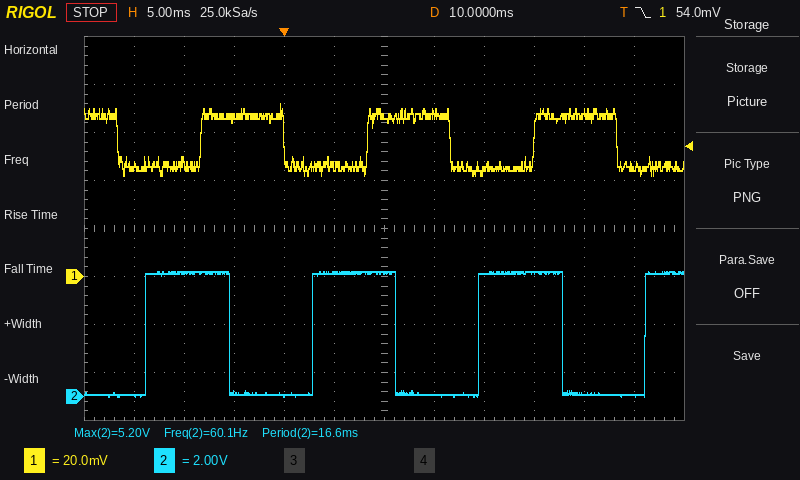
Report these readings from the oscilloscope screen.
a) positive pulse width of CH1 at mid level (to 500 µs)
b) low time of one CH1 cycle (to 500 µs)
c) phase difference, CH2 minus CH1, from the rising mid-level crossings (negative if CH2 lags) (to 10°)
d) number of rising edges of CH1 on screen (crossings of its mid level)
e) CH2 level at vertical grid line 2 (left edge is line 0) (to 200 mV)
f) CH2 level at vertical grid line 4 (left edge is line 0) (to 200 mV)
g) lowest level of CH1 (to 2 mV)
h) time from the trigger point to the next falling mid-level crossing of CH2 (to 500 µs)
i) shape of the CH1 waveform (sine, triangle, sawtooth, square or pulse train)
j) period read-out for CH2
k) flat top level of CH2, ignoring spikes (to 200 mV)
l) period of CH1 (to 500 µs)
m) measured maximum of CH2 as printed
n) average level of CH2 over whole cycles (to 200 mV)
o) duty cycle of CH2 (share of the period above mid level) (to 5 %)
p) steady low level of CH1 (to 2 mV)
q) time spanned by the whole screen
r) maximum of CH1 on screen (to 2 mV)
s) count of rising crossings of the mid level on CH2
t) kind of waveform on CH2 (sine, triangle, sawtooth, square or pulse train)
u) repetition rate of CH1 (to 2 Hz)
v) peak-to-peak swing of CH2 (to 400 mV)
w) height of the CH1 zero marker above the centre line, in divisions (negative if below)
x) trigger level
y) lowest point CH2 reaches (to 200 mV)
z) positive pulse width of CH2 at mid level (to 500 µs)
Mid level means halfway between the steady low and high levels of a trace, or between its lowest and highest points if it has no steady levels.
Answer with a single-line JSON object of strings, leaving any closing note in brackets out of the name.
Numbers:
{"positive pulse width of CH1 at mid level": "8.5 ms", "low time of one CH1 cycle": "8.5 ms", "phase difference, CH2 minus CH1, from the rising mid-level crossings (negative if CH2 lags)": "+120°", "number of rising edges of CH1 on screen": "3", "CH2 level at vertical grid line 2 (left edge is line 0)": "5.2 V", "CH2 level at vertical grid line 4 (left edge is line 0)": "0.0 V", "lowest level of CH1": "42 mV", "time from the trigger point to the next falling mid-level crossing of CH2": "11.0 ms", "shape of the CH1 waveform": "square", "period read-out for CH2": "16.6 ms", "flat top level of CH2, ignoring spikes": "5.2 V", "period of CH1": "16.5 ms", "measured maximum of CH2 as printed": "5.20 V", "average level of CH2 over whole cycles": "2.6 V", "duty cycle of CH2 (share of the period above mid level)": "50 %", "steady low level of CH1": "46 mV", "time spanned by the whole screen": "60 ms", "maximum of CH1 on screen": "72 mV", "count of rising crossings of the mid level on CH2": "4", "kind of waveform on CH2": "square", "repetition rate of CH1": "60 Hz", "peak-to-peak swing of CH2": "5.2 V", "height of the CH1 zero marker above the centre line, in divisions": "-1.0 div", "trigger level": "54.0 mV", "lowest point CH2 reaches": "0.0 V", "positive pulse width of CH2 at mid level": "8.5 ms"}
